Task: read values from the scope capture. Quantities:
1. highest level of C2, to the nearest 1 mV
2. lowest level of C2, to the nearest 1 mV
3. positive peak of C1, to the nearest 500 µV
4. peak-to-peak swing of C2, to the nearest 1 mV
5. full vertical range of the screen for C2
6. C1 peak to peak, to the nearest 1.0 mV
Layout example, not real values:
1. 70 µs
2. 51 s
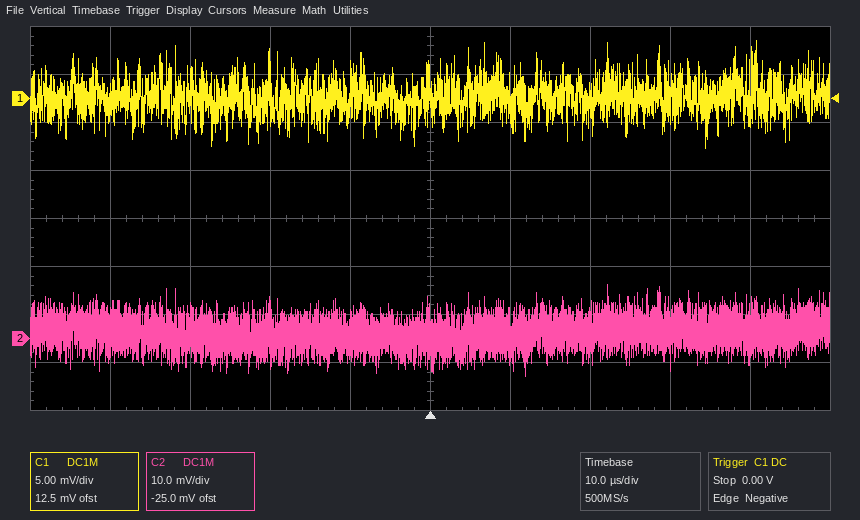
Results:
1. 11 mV
2. -8 mV
3. 6.0 mV
4. 19 mV
5. 80 mV
6. 11.0 mV
